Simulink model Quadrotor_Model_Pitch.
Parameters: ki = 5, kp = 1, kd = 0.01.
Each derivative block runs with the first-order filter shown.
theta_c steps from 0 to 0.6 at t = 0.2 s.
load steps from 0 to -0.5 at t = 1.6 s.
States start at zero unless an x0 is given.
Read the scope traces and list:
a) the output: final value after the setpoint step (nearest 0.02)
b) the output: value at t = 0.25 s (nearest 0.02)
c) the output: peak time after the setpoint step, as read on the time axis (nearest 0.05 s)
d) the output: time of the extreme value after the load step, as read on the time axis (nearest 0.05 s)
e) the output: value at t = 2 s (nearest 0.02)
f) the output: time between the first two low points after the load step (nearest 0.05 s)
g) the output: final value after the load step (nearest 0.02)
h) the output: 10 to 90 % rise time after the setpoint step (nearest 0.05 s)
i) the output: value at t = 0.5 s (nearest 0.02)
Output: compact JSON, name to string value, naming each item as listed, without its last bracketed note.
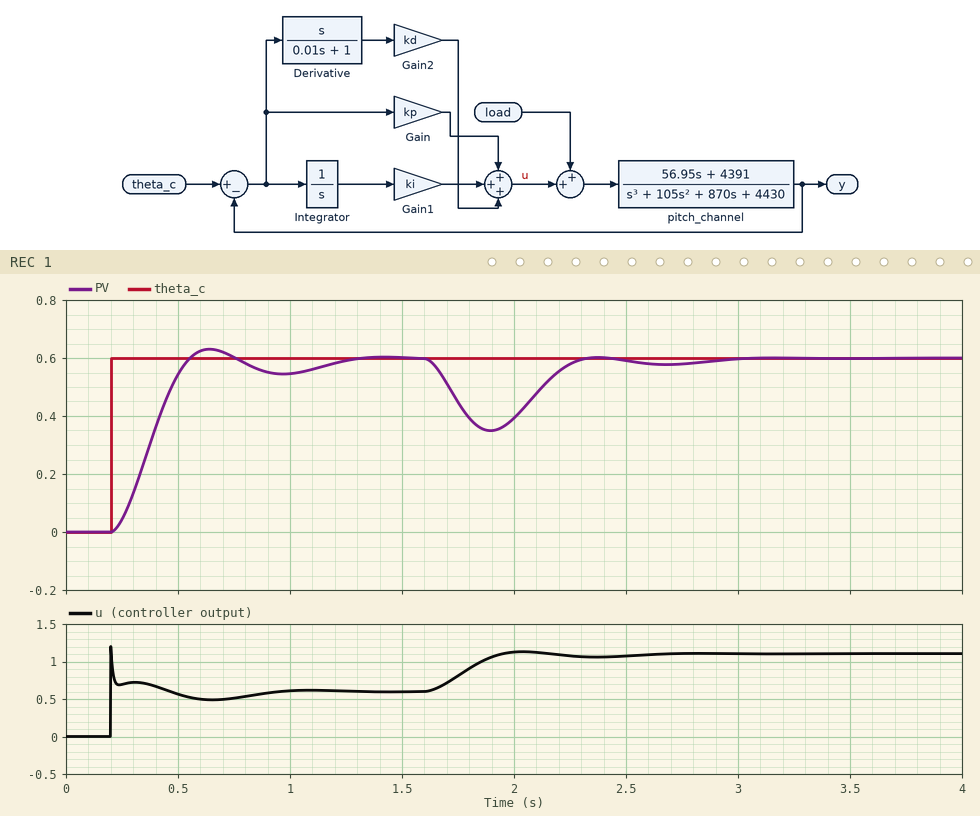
{"the output: final value after the setpoint step": "0.60", "the output: value at t = 0.25 s": "0.04", "the output: peak time after the setpoint step, as read on the time axis": "0.65 s", "the output: time of the extreme value after the load step, as read on the time axis": "1.90 s", "the output: value at t = 2 s": "0.40", "the output: time between the first two low points after the load step": "0.80 s", "the output: final value after the load step": "0.60", "the output: 10 to 90 % rise time after the setpoint step": "0.25 s", "the output: value at t = 0.5 s": "0.54"}
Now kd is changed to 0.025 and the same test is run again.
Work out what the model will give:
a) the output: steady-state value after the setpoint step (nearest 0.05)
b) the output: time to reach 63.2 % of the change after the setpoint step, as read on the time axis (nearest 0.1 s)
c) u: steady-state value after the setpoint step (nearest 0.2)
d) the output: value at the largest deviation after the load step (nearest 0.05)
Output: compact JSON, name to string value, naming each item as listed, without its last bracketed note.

{"the output: steady-state value after the setpoint step": "0.60", "the output: time to reach 63.2 % of the change after the setpoint step, as read on the time axis": "0.4 s", "u: steady-state value after the setpoint step": "0.6", "the output: value at the largest deviation after the load step": "0.35"}
